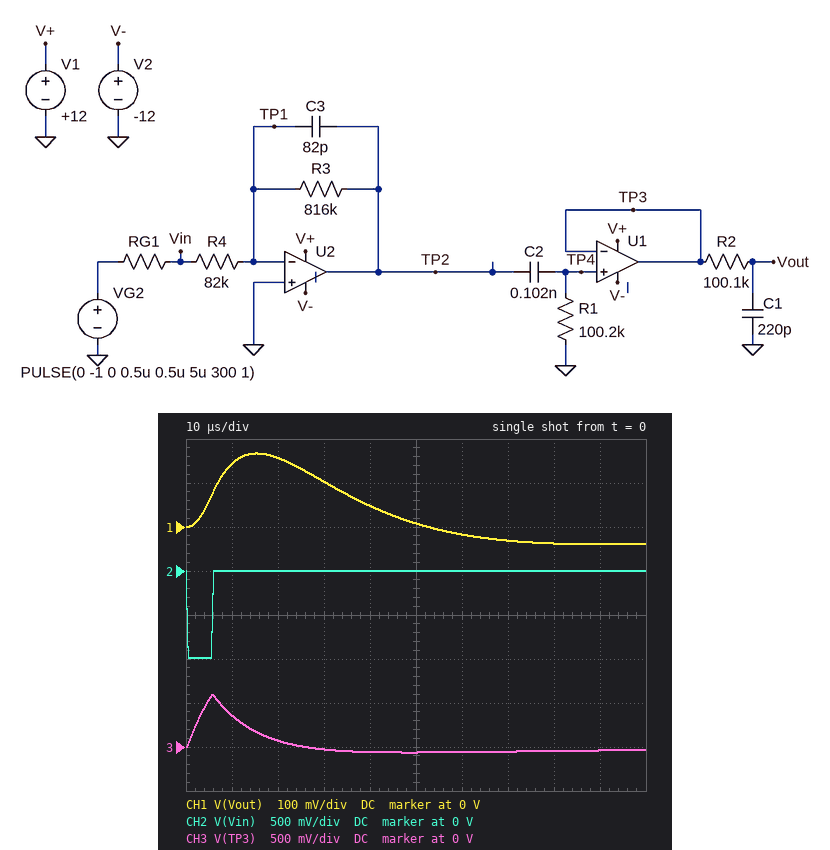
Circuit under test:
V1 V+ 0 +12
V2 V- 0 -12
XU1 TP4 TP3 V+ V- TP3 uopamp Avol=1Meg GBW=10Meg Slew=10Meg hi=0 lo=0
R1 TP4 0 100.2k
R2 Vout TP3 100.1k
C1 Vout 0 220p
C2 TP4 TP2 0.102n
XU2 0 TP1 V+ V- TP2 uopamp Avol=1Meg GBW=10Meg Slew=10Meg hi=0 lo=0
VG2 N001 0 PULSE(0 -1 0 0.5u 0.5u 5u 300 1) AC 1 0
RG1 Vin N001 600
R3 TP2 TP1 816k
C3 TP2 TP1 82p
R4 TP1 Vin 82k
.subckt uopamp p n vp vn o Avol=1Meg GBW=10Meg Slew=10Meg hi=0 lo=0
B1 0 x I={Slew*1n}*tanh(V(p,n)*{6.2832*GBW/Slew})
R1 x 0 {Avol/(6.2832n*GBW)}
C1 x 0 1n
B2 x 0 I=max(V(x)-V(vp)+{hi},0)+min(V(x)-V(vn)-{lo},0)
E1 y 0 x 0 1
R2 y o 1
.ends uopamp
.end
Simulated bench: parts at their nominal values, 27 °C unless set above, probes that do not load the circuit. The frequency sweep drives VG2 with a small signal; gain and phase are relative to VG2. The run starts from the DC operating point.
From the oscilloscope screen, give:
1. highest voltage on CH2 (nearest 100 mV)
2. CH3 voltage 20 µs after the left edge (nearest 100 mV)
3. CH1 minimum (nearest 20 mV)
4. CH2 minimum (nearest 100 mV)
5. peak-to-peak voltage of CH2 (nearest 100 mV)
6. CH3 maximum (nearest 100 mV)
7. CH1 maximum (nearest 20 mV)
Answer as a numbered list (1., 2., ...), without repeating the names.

1. 0 V
2. 100 mV
3. -40 mV
4. -1.0 V
5. 1.0 V
6. 600 mV
7. 160 mV
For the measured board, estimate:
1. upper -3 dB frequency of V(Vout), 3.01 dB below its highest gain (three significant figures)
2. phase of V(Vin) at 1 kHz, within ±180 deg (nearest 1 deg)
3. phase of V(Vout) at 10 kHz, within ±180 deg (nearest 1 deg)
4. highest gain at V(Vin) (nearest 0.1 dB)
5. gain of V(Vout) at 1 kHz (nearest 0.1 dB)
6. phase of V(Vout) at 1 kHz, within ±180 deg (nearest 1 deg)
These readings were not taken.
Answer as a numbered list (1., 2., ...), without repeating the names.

1. 9.18 kHz
2. 0 deg
3. 106 deg
4. -0.1 dB
5. -4.8 dB
6. -124 deg
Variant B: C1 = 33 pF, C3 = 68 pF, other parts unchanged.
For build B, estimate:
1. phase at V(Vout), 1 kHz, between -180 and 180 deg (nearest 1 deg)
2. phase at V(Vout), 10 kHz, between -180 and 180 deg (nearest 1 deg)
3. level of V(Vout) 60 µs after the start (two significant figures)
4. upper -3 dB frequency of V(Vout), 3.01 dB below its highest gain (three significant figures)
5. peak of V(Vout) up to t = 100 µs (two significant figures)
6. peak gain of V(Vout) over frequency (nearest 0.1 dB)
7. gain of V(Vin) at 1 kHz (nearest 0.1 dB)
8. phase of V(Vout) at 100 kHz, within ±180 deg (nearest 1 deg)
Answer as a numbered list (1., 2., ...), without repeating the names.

1. -114 deg
2. 151 deg
3. -77 mV
4. 18.6 kHz
5. 510 mV
6. 3.6 dB
7. -0.1 dB
8. 35 deg
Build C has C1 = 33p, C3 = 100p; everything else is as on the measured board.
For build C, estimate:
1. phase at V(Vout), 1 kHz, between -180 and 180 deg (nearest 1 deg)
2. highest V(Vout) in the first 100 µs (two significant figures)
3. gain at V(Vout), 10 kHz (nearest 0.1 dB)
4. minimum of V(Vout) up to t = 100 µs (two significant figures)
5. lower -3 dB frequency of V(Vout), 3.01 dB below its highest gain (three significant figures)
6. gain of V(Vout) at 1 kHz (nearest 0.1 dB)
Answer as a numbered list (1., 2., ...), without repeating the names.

1. -122 deg
2. 350 mV
3. 0 dB
4. -45 mV
5. 1.57 kHz
6. -5.0 dB
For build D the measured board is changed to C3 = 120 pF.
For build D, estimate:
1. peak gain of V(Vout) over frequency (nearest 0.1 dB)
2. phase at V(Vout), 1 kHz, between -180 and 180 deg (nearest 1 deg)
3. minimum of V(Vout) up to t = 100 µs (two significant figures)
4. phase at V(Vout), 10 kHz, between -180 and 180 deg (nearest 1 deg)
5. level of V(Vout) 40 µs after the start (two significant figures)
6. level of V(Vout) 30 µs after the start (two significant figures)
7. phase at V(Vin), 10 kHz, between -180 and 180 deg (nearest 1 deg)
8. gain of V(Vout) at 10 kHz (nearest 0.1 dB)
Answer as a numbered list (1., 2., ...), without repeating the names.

1. -1.7 dB
2. -133 deg
3. -23 mV
4. 102 deg
5. 44 mV
6. 80 mV
7. 0 deg
8. -6.0 dB
